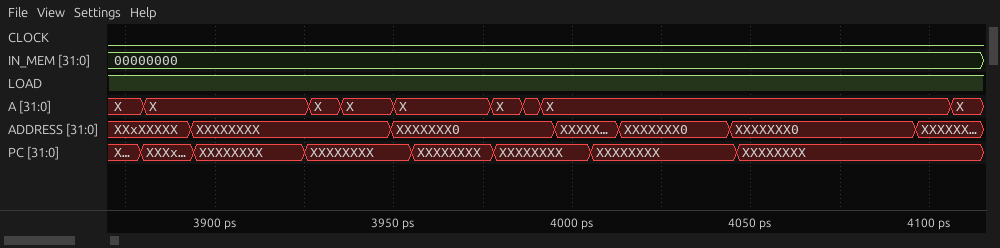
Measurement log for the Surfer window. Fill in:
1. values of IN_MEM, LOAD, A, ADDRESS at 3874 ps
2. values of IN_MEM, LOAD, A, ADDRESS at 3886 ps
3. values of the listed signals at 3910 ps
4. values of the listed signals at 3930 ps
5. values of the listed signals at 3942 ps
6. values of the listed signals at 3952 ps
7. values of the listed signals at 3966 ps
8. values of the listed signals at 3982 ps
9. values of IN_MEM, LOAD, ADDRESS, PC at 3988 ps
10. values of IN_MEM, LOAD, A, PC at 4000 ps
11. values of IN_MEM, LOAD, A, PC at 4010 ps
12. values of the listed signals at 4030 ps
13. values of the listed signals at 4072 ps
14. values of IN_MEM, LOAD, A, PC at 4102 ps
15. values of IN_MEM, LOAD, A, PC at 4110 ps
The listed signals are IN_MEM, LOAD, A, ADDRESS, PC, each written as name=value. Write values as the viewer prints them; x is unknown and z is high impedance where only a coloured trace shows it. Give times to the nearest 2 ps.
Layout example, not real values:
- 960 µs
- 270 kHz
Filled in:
- IN_MEM=00000000, LOAD=1, A=X, ADDRESS=XXxXXXXX
- IN_MEM=00000000, LOAD=1, A=X, ADDRESS=XXxXXXXX
- IN_MEM=00000000, LOAD=1, A=X, ADDRESS=XXXXXXXX, PC=XXXXXXXX
- IN_MEM=00000000, LOAD=1, A=X, ADDRESS=XXXXXXXX, PC=XXXXXXXX
- IN_MEM=00000000, LOAD=1, A=X, ADDRESS=XXXXXXXX, PC=XXXXXXXX
- IN_MEM=00000000, LOAD=1, A=X, ADDRESS=XXXXXXX0, PC=XXXXXXXX
- IN_MEM=00000000, LOAD=1, A=X, ADDRESS=XXXXXXX0, PC=XXXXXXXX
- IN_MEM=00000000, LOAD=1, A=X, ADDRESS=XXXXXXX0, PC=XXXXXXXX
- IN_MEM=00000000, LOAD=1, ADDRESS=XXXXXXX0, PC=XXXXXXXX
- IN_MEM=00000000, LOAD=1, A=X, PC=XXXXXXXX
- IN_MEM=00000000, LOAD=1, A=X, PC=XXXXXXXX
- IN_MEM=00000000, LOAD=1, A=X, ADDRESS=XXXXXXX0, PC=XXXXXXXX
- IN_MEM=00000000, LOAD=1, A=X, ADDRESS=XXXXXXX0, PC=XXXXXXXX
- IN_MEM=00000000, LOAD=1, A=X, PC=XXXXXXXX
- IN_MEM=00000000, LOAD=1, A=X, PC=XXXXXXXX
